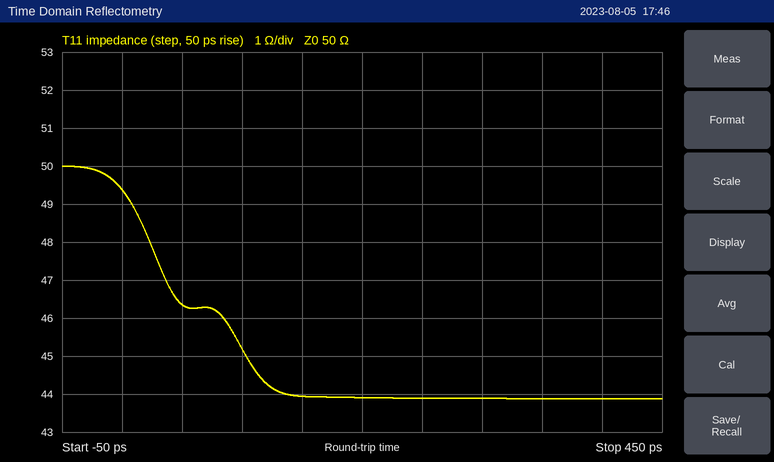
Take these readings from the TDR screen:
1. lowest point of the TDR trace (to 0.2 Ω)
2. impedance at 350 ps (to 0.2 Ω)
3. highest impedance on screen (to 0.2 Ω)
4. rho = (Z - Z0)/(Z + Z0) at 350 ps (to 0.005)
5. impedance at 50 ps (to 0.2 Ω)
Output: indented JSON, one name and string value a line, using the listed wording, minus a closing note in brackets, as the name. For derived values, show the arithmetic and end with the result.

{
  "lowest point of the TDR trace": "43.8 Ω",
  "impedance at 350 ps": "43.8 Ω",
  "highest impedance on screen": "50.0 Ω",
  "rho = (Z - Z0)/(Z + Z0) at 350 ps": "(43.8 − 50)/(43.8 + 50) ≈ -0.0661, so -0.065 to the nearest 0.005",
  "impedance at 50 ps": "46.4 Ω"
}
